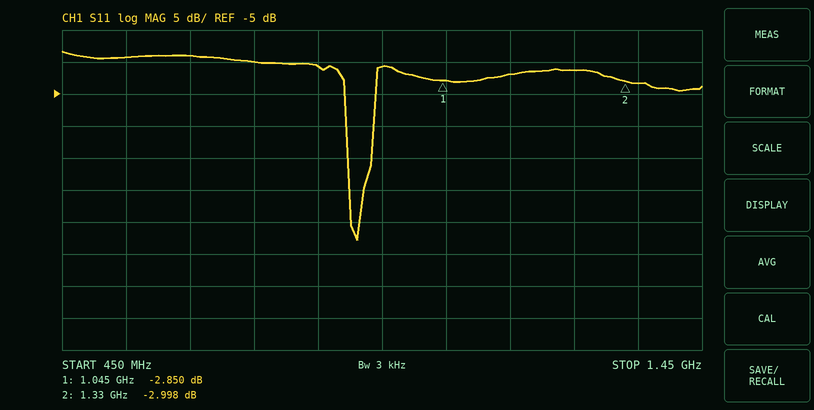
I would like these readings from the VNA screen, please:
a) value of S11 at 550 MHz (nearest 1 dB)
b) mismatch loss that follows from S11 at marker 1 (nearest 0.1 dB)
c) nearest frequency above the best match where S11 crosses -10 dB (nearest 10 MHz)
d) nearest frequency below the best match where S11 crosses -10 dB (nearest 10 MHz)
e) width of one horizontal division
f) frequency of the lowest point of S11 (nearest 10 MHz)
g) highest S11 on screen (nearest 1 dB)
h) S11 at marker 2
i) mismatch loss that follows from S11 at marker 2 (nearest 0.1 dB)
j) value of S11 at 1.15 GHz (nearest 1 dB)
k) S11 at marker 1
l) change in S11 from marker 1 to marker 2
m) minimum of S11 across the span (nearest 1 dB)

1 dB
3.2 dB
940 MHz
890 MHz
100 MHz
910 MHz
2 dB
-2.998 dB
3.0 dB
-2 dB
-2.850 dB
-0.148 dB
-28 dB
